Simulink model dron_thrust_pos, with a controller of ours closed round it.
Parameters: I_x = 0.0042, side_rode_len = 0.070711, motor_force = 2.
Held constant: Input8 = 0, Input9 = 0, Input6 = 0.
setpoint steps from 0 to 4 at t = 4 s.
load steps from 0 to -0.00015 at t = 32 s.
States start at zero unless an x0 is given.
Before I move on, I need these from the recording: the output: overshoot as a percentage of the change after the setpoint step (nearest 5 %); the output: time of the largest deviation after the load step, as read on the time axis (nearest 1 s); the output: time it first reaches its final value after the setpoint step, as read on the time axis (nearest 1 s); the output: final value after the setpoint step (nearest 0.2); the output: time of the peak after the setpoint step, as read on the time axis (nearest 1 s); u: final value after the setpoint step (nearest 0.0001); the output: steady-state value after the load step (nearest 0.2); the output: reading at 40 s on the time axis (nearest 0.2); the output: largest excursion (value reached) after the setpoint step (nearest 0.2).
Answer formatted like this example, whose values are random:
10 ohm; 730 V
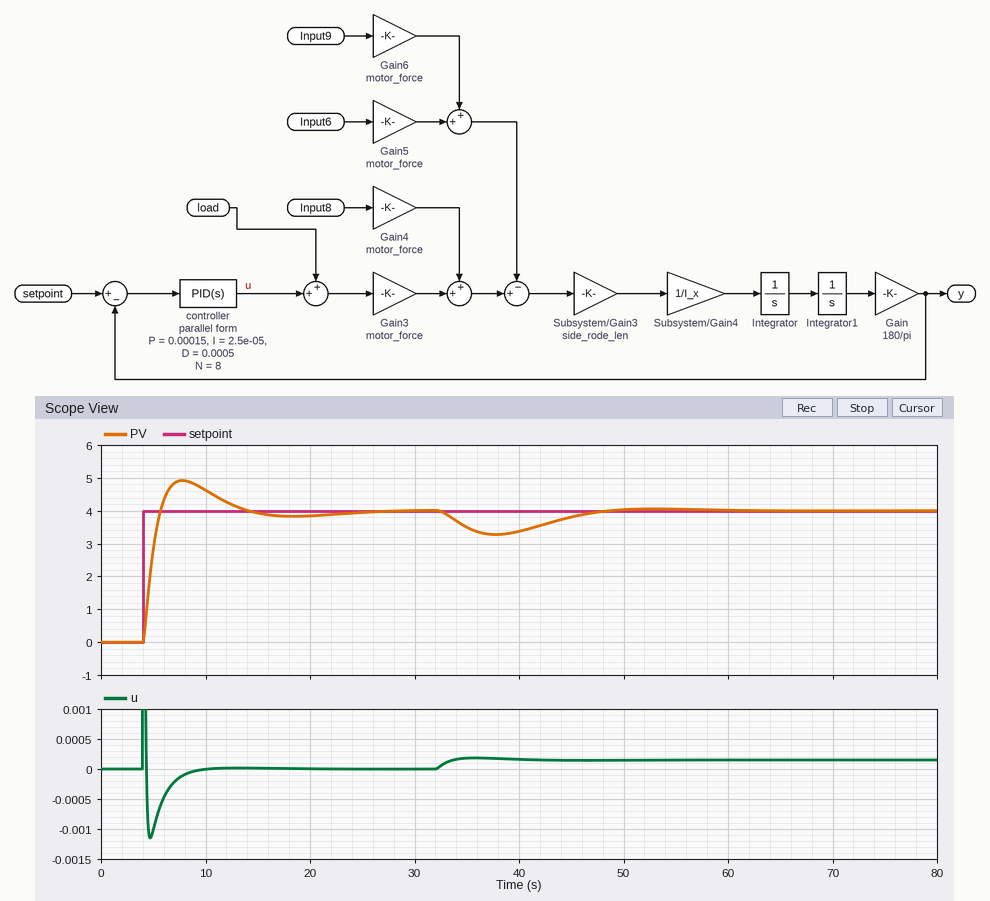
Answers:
25 %; 38 s; 6 s; 4.0; 8 s; 0.0000; 4.0; 3.4; 5.0
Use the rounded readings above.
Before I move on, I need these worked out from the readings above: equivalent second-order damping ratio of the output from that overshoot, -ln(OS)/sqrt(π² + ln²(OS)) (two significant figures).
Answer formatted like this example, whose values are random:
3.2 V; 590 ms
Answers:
0.40
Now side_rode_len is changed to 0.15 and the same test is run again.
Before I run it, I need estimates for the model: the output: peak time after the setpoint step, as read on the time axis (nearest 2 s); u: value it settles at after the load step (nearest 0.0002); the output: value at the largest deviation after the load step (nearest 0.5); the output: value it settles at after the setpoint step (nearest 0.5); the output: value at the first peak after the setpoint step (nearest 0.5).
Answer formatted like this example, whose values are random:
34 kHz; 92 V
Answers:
6 s; 0.0002; 3.5; 4.0; 4.5
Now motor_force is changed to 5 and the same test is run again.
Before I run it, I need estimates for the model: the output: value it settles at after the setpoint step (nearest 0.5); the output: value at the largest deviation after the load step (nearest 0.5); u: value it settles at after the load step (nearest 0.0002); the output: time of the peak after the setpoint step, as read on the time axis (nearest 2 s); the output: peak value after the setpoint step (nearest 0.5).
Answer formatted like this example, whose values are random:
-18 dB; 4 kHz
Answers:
4.0; 3.5; 0.0002; 6 s; 4.5
